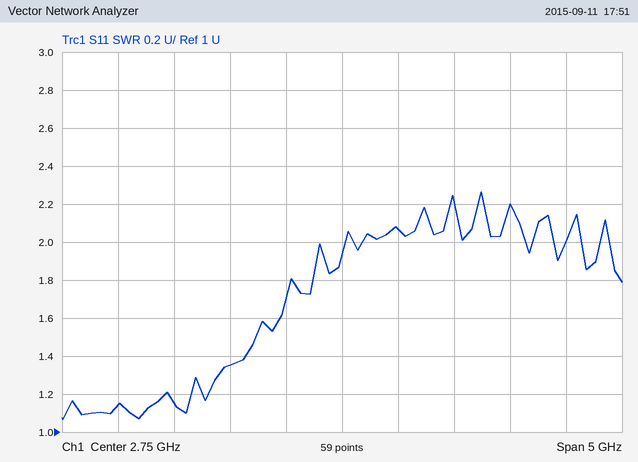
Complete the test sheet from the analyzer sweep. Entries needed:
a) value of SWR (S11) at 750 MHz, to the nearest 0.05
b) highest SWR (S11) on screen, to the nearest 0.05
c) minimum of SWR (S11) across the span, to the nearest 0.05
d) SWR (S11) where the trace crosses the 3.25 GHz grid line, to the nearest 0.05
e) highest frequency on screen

1.15
2.25
1.05
2.05
5.25 GHz
